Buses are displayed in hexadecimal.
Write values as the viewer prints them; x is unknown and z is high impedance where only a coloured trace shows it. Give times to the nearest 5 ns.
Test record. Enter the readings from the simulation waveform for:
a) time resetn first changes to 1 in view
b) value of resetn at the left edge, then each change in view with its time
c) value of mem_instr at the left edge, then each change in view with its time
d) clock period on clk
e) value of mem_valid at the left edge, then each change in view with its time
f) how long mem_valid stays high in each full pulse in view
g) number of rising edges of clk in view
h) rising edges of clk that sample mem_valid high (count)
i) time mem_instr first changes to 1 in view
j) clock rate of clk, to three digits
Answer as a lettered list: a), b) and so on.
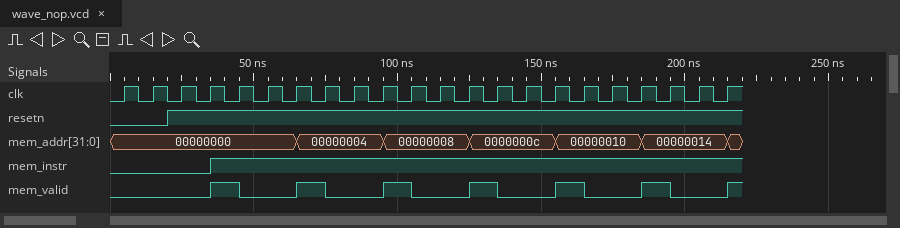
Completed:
a) 20 ns
b) 0, 1 at 20 ns
c) 0, 1 at 35 ns
d) 10 ns
e) 0, 1 at 35 ns, 0 at 45 ns, 1 at 65 ns, 0 at 75 ns, 1 at 95 ns, 0 at 105 ns, 1 at 125 ns, 0 at 135 ns, 1 at 155 ns, 0 at 165 ns, 1 at 185 ns, 0 at 195 ns, 1 at 215 ns
f) 10 ns, 10 ns, 10 ns, 10 ns, 10 ns, 10 ns
g) 22
h) 6
i) 35 ns
j) 100 MHz
